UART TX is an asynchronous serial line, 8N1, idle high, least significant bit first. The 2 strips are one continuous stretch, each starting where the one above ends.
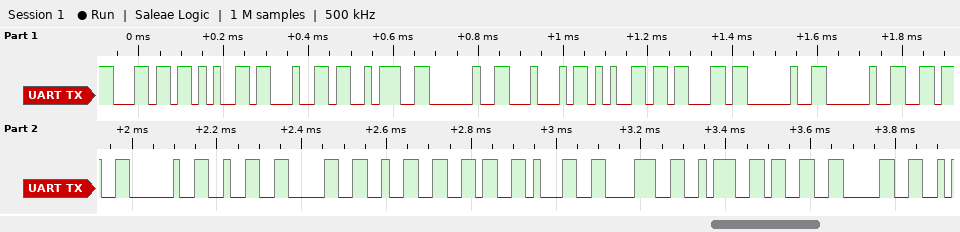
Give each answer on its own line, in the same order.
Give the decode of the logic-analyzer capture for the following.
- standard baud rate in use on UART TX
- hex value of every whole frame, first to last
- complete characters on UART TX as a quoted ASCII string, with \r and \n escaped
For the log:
57600 baud
6C 65 64 3A 20 44 65 63 20 20 36 20 32 30 32 36 31 38 3A 33 30
"led: Dec  6 202618:30"
